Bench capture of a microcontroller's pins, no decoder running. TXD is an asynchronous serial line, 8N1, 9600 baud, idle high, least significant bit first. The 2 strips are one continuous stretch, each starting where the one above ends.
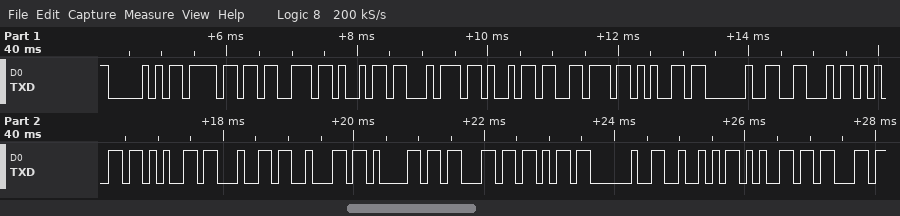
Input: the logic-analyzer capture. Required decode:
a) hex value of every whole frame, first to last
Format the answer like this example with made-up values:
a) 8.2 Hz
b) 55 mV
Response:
a) 50 6F 73 69 74 69 76 65 20 46 65 65 64 62 61 63 6B 20 52 65 63
